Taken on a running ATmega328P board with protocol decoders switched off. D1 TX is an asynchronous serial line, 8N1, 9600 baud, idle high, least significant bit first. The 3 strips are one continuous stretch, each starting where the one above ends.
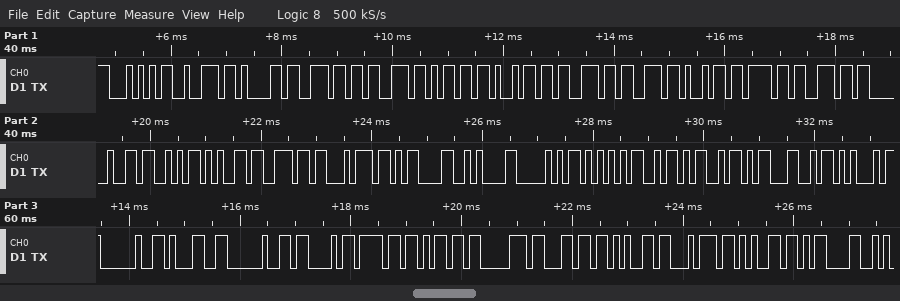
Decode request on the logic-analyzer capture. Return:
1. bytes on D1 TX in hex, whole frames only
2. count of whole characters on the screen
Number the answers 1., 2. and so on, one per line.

1. 0x54 0x72 0x61 0x6E 0x73 0x6D 0x69 0x73 0x73 0x69 0x6F 0x6E 0x20 0x53 0x65 0x6E 0x74 0x0D 0x0A 0x50 0x55 0x5A 0x5A 0x4C 0x45 0x20 0x31 0x20 0x43 0x6F 0x6D 0x70 0x6C 0x65 0x74 0x65 0x0D
2. 37
